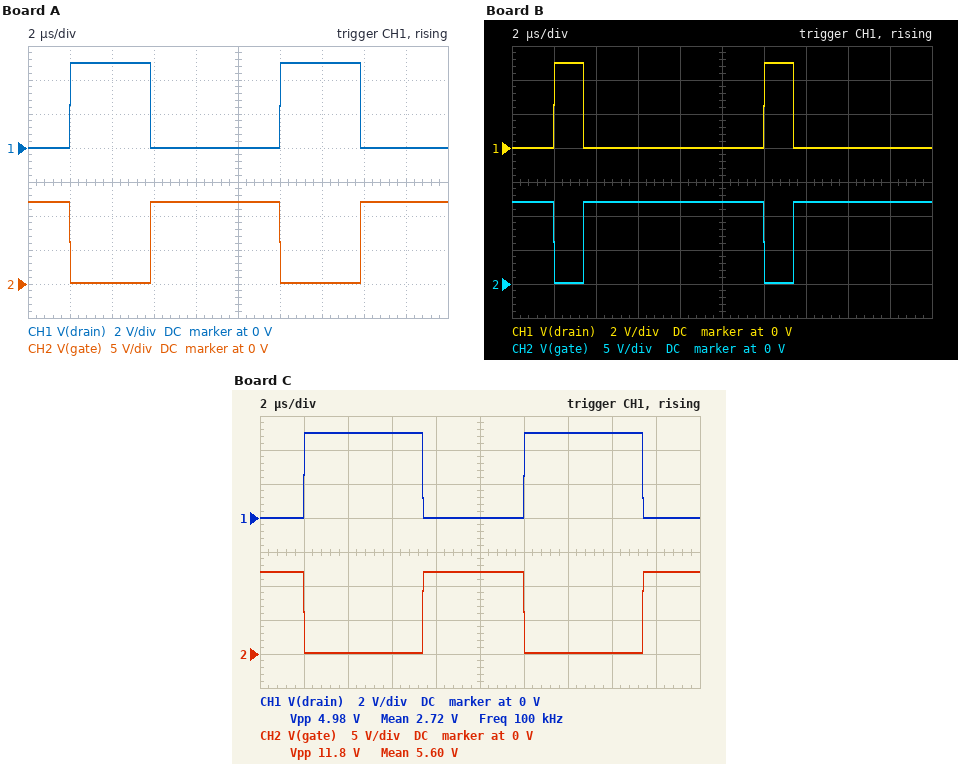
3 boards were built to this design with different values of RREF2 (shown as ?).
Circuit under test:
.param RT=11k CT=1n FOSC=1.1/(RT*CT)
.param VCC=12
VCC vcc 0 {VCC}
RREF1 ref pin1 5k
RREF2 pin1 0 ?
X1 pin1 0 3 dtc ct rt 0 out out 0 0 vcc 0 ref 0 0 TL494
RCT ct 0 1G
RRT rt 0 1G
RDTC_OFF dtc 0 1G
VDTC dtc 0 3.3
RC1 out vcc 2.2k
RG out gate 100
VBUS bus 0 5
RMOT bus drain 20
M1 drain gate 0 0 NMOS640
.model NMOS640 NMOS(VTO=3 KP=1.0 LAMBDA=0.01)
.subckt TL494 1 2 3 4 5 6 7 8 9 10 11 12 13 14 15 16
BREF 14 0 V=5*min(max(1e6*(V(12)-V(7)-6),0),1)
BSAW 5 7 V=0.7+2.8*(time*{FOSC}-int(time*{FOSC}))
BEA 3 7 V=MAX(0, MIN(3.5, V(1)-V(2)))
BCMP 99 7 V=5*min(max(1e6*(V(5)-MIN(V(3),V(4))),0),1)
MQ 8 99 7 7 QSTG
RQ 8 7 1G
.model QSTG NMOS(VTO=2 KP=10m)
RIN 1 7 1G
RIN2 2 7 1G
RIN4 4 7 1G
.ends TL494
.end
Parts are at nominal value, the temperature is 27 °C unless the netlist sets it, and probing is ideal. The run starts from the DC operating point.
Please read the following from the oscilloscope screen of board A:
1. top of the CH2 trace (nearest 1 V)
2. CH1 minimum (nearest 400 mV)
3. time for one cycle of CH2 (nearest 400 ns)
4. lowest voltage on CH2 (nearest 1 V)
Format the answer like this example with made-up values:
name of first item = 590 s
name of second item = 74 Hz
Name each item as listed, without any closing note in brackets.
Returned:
top of the CH2 trace = 12 V
CH1 minimum = 0 V
time for one cycle of CH2 = 10.0 µs
lowest voltage on CH2 = 0 V
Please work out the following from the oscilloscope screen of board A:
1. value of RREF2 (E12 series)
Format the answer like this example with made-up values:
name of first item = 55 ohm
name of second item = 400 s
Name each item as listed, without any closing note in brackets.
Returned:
value of RREF2 = 4.7 kΩ
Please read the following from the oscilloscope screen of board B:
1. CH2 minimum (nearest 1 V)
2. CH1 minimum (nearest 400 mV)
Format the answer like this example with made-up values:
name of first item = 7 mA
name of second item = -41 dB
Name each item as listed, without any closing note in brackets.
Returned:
CH2 minimum = 0 V
CH1 minimum = 0 V
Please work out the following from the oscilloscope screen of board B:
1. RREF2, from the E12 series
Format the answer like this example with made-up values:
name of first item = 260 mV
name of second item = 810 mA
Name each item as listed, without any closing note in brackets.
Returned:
RREF2, from the E12 series = 8.2 kΩ
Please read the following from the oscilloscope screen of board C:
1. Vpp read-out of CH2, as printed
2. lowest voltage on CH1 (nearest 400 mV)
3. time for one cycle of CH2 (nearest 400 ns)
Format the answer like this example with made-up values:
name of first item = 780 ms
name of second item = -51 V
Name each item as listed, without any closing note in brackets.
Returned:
Vpp read-out of CH2, as printed = 11.8 V
lowest voltage on CH1 = 0 V
time for one cycle of CH2 = 10.0 µs
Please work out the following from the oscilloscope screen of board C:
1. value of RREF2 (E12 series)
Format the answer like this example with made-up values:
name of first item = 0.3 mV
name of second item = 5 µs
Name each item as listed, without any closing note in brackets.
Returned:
value of RREF2 = 3.3 kΩ
